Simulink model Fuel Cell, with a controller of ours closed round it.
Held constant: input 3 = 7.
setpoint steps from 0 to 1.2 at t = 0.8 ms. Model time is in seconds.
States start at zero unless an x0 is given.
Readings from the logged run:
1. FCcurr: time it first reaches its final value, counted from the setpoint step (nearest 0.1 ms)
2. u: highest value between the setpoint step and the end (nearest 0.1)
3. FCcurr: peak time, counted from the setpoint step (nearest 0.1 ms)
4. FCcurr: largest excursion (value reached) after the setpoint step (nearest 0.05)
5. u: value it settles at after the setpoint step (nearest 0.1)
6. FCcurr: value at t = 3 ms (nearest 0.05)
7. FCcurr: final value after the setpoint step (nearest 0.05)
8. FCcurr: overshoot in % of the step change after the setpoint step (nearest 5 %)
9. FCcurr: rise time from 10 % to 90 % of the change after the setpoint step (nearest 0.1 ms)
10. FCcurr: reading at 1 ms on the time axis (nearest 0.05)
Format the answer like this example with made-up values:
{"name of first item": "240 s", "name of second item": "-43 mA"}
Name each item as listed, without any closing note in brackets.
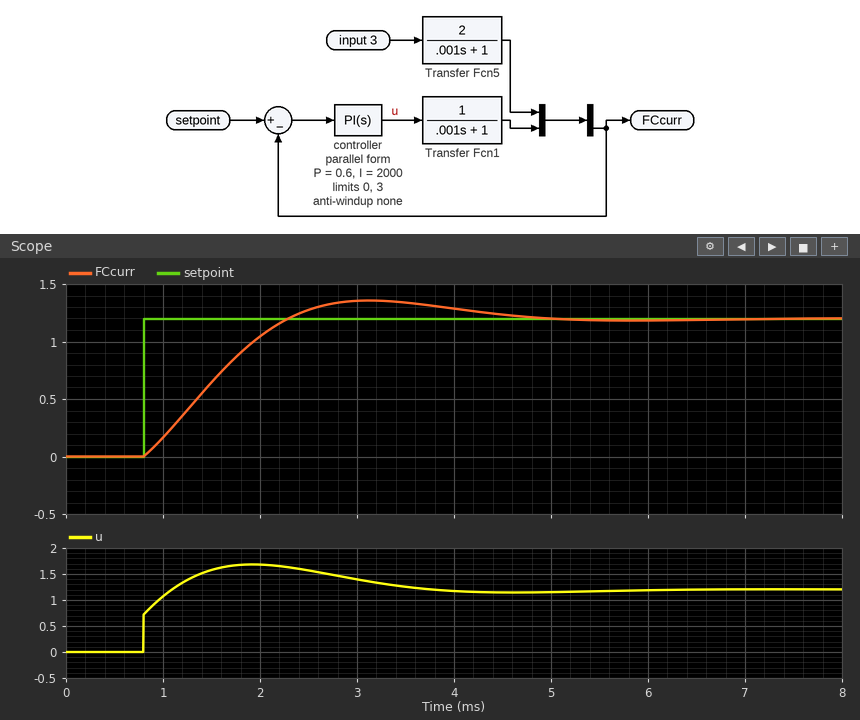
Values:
{"FCcurr: time it first reaches its final value, counted from the setpoint step": "1.5 ms", "u: highest value between the setpoint step and the end": "1.7", "FCcurr: peak time, counted from the setpoint step": "2.3 ms", "FCcurr: largest excursion (value reached) after the setpoint step": "1.35", "u: value it settles at after the setpoint step": "1.2", "FCcurr: value at t = 3 ms": "1.35", "FCcurr: final value after the setpoint step": "1.20", "FCcurr: overshoot in % of the step change after the setpoint step": "15 %", "FCcurr: rise time from 10 % to 90 % of the change after the setpoint step": "1.1 ms", "FCcurr: reading at 1 ms on the time axis": "0.15"}
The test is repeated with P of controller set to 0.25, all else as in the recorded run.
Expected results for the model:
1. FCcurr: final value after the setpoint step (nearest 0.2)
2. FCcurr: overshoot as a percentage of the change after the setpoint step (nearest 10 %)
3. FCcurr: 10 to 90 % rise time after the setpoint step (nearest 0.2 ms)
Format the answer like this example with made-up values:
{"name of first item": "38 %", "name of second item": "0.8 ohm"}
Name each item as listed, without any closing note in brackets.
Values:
{"FCcurr: final value after the setpoint step": "1.2", "FCcurr: overshoot as a percentage of the change after the setpoint step": "20 %", "FCcurr: 10 to 90 % rise time after the setpoint step": "1.0 ms"}
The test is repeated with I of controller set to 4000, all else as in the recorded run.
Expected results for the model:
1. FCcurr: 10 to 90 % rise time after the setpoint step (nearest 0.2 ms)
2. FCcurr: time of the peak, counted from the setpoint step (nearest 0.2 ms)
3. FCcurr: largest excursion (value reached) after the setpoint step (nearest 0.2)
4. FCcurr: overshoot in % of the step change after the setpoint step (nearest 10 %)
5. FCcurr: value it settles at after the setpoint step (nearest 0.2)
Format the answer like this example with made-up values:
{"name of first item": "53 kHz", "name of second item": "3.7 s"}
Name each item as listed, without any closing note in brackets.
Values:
{"FCcurr: 10 to 90 % rise time after the setpoint step": "0.6 ms", "FCcurr: time of the peak, counted from the setpoint step": "1.6 ms", "FCcurr: largest excursion (value reached) after the setpoint step": "1.6", "FCcurr: overshoot in % of the step change after the setpoint step": "30 %", "FCcurr: value it settles at after the setpoint step": "1.2"}
